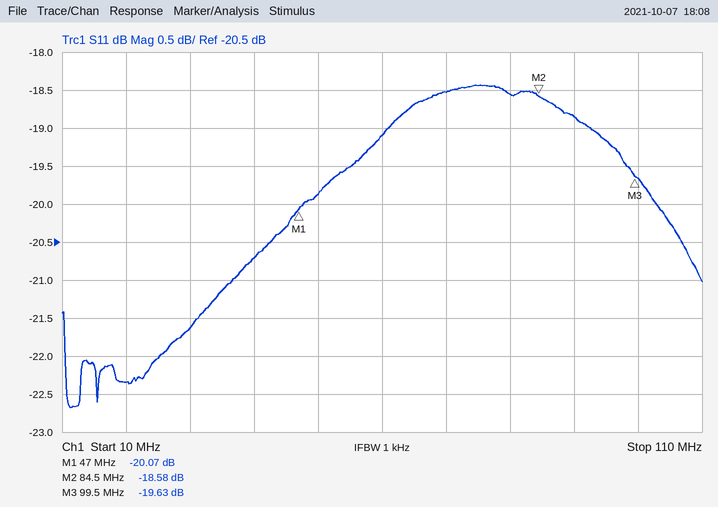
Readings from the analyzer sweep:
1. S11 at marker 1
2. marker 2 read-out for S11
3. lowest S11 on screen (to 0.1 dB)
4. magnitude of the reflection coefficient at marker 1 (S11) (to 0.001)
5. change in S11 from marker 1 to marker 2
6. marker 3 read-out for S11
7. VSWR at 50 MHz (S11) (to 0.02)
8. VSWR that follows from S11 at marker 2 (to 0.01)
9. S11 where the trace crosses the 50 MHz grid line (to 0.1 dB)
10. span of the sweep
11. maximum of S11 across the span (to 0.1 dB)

-20.07 dB
-18.58 dB
-22.7 dB
0.099
1.49 dB
-19.63 dB
1.22
1.27
-19.9 dB
100 MHz
-18.4 dB
